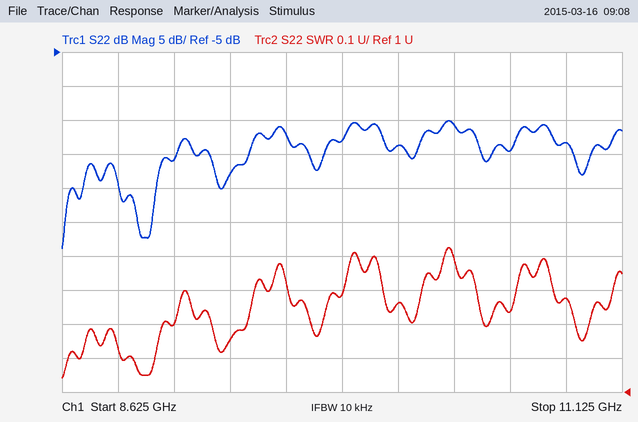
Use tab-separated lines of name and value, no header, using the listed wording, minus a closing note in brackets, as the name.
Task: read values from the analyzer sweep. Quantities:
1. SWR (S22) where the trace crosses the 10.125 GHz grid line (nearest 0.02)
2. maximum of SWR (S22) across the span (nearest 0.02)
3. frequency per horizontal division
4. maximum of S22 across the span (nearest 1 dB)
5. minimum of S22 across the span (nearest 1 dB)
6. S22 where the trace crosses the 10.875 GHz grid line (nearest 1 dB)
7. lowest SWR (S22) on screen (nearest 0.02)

SWR (S22) where the trace crosses the 10.125 GHz grid line	1.26
maximum of SWR (S22) across the span	1.42
frequency per horizontal division	250 MHz
maximum of S22 across the span	-15 dB
minimum of S22 across the span	-34 dB
S22 where the trace crosses the 10.875 GHz grid line	-18 dB
lowest SWR (S22) on screen	1.04
